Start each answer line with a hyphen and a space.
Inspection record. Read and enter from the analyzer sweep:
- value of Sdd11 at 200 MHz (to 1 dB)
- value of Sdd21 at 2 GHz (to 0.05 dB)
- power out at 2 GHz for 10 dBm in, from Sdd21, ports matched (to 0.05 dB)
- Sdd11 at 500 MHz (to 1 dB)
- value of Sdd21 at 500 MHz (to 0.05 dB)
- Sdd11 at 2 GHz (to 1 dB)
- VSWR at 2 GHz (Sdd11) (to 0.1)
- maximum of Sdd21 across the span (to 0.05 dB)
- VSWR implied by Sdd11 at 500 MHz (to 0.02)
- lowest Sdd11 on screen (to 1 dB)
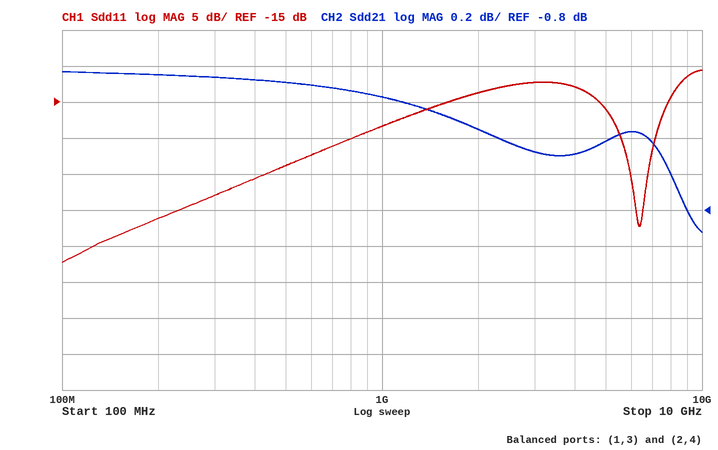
- -31 dB
- -0.35 dB
- 9.65 dBm
- -24 dB
- -0.10 dB
- -14 dB
- 1.5
- -0.05 dB
- 1.14
- -37 dB
